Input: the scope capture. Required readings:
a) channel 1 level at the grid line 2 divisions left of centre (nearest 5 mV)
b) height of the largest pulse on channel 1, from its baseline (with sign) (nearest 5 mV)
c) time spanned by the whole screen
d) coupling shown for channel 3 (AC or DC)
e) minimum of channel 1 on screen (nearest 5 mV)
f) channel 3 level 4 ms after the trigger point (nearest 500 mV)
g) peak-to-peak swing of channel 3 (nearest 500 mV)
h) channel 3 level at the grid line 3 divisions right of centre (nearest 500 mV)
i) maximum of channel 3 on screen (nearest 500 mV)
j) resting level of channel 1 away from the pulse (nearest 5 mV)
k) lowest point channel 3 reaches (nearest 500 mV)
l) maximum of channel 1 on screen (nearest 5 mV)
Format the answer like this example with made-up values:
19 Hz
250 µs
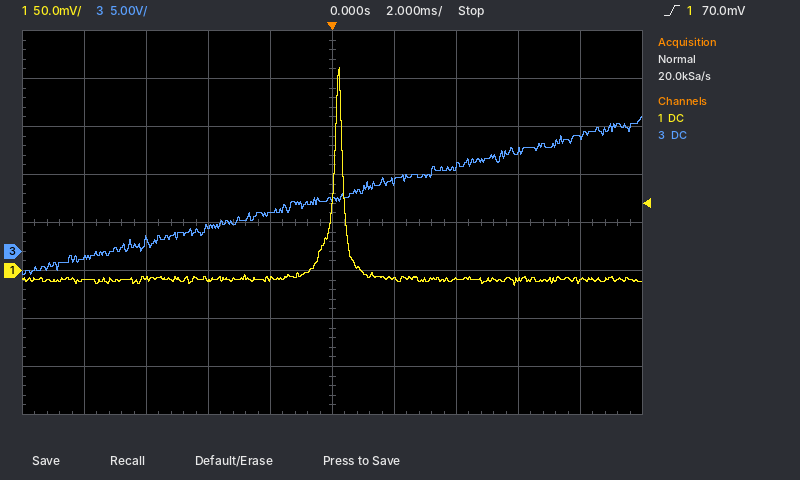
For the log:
-10 mV
+220 mV
20 ms
DC
-15 mV
9.0 V
16.5 V
10.5 V
14.0 V
-10 mV
-2.5 V
210 mV
